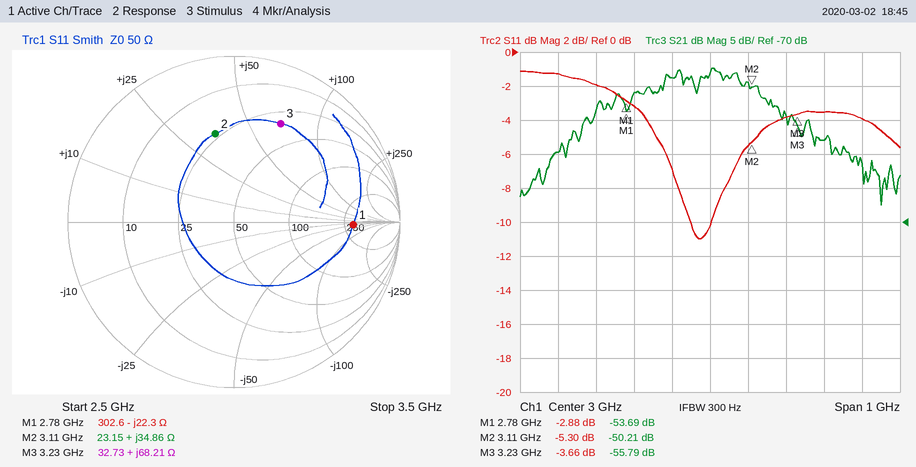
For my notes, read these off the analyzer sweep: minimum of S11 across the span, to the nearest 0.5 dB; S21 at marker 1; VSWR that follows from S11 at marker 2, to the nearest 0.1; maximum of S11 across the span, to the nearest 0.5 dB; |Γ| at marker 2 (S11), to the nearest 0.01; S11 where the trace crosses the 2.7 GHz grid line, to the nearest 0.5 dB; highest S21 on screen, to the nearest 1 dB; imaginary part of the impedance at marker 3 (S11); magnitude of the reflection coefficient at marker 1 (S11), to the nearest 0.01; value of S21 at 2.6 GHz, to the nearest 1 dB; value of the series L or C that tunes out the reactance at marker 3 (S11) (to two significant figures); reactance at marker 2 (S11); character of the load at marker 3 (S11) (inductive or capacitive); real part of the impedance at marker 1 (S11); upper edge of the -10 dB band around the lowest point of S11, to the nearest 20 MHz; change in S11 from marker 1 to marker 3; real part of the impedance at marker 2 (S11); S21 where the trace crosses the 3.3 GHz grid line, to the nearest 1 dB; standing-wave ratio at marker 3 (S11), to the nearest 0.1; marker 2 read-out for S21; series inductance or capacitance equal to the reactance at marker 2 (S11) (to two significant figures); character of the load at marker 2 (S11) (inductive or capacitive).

-11.0 dB
-53.69 dB
3.4
-1.0 dB
0.54
-2.0 dB
-47 dB
+68.21 Ω
0.72
-60 dB
720 fF
+34.86 Ω
inductive
302.6 Ω
3.00 GHz
-0.78 dB
23.15 Ω
-58 dB
4.8
-50.21 dB
1.8 nH
inductive
